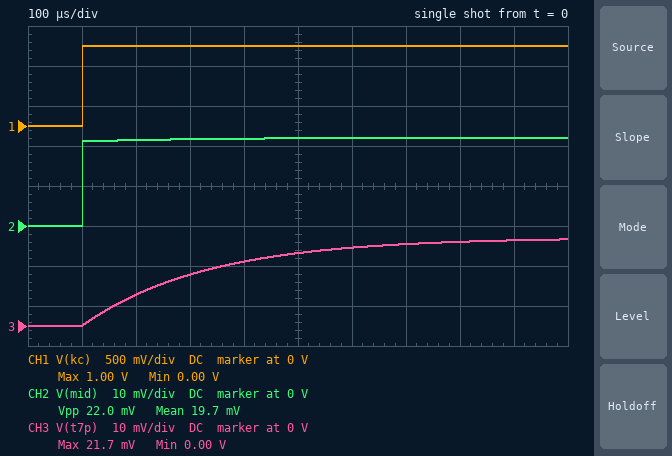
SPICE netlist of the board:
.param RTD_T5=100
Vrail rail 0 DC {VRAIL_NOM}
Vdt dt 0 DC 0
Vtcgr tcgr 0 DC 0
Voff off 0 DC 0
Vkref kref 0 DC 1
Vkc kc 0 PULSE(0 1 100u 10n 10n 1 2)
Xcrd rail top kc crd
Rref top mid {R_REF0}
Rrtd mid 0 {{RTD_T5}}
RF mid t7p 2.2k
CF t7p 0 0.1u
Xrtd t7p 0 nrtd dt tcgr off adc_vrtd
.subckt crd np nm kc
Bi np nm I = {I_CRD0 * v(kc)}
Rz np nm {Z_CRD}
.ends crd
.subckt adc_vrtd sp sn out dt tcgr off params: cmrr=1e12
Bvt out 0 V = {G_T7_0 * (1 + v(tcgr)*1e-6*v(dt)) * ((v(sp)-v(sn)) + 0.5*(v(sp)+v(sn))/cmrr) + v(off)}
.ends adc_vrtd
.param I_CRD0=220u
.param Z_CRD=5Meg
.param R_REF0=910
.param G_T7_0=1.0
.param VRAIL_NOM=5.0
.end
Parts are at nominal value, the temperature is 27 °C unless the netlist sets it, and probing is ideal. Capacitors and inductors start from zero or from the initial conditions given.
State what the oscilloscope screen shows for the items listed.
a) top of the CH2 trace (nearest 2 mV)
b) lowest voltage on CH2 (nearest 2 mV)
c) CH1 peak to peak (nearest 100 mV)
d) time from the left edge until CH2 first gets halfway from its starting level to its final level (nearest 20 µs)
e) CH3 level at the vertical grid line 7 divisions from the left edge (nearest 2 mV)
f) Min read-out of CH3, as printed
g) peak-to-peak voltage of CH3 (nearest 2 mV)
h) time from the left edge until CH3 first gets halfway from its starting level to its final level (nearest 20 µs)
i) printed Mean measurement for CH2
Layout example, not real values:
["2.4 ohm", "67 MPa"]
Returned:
["22 mV", "0 V", "1.0 V", "100 µs", "20 mV", "0.00 V", "22 mV", "260 µs", "19.7 mV"]
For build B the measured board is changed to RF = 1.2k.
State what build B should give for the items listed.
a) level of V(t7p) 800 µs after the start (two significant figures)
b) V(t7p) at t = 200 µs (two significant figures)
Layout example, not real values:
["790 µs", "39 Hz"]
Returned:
["22 mV", "12 mV"]
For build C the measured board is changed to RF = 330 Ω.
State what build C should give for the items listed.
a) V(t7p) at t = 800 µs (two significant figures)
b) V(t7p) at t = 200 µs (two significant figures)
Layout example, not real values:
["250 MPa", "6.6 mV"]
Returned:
["22 mV", "20 mV"]
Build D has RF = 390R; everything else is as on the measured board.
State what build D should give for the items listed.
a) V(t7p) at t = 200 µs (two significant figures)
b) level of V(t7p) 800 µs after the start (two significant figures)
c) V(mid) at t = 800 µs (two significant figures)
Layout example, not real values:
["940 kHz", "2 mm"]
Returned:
["19 mV", "22 mV", "22 mV"]
